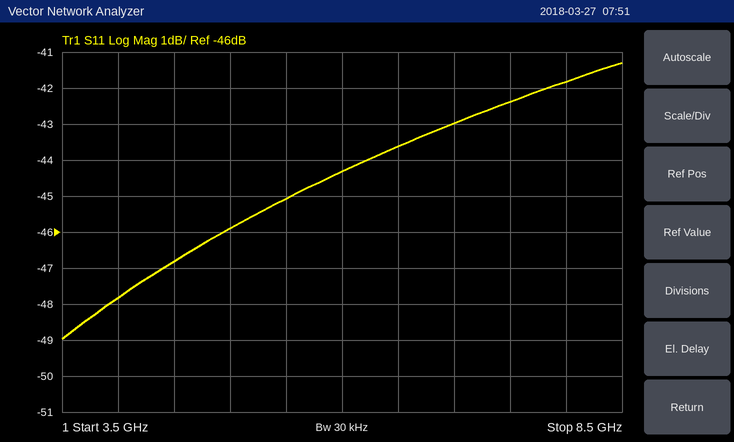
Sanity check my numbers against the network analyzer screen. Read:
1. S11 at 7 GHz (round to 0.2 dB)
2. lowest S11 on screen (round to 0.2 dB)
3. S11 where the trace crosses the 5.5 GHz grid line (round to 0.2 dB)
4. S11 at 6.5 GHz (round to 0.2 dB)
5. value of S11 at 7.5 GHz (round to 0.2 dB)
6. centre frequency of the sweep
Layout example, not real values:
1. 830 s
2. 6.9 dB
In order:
1. -43.0 dB
2. -49.0 dB
3. -45.0 dB
4. -43.6 dB
5. -42.4 dB
6. 6 GHz
